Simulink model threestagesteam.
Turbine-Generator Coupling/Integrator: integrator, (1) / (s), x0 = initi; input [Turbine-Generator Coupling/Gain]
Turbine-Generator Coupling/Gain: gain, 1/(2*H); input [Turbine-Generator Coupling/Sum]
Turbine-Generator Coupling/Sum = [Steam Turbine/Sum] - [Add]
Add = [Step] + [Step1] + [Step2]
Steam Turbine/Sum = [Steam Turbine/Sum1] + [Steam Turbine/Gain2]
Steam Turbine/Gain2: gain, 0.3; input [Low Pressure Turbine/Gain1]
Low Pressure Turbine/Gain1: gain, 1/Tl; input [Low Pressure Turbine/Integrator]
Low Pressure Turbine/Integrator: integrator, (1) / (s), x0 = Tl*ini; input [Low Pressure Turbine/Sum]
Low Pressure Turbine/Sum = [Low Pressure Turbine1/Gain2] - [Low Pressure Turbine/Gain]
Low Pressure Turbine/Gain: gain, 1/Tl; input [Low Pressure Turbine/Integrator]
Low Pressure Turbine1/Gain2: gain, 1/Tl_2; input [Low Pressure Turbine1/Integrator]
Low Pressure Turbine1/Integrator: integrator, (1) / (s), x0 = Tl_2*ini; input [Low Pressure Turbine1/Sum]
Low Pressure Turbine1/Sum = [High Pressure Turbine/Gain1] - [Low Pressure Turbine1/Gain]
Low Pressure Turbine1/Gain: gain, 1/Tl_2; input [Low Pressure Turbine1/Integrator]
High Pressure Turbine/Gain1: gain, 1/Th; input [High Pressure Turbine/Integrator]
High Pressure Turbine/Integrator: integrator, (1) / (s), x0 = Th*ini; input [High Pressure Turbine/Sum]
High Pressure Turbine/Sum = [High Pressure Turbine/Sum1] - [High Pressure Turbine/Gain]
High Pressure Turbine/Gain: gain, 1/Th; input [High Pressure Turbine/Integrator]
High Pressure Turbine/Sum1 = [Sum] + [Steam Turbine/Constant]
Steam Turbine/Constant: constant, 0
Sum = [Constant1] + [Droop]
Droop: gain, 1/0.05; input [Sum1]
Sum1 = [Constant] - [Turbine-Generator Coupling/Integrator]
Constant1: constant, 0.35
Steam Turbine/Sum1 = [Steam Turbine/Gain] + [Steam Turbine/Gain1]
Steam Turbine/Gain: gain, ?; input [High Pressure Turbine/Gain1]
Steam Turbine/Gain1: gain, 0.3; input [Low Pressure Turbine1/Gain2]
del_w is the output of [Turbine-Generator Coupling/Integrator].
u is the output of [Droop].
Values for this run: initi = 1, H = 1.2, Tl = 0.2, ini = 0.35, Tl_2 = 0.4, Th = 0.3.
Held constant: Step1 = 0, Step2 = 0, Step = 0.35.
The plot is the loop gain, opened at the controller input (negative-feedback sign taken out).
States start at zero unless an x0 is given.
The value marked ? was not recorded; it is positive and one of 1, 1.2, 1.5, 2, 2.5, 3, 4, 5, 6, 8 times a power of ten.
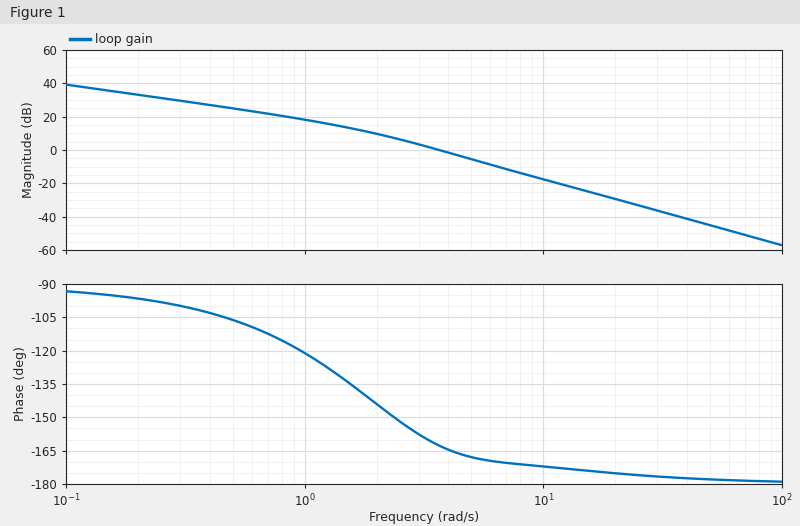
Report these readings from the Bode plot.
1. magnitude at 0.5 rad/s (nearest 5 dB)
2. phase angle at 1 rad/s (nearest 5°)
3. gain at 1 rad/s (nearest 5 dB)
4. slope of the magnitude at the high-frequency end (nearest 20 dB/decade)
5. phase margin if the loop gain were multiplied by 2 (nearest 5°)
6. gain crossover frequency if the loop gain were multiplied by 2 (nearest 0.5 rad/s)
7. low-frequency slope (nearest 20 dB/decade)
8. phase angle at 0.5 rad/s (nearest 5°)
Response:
25 dB
-120°
20 dB
-40 dB/decade
10°
5.0 rad/s
-20 dB/decade
-105°
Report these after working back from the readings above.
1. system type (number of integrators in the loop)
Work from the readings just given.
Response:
1
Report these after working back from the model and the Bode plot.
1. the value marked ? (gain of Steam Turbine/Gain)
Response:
0.5
